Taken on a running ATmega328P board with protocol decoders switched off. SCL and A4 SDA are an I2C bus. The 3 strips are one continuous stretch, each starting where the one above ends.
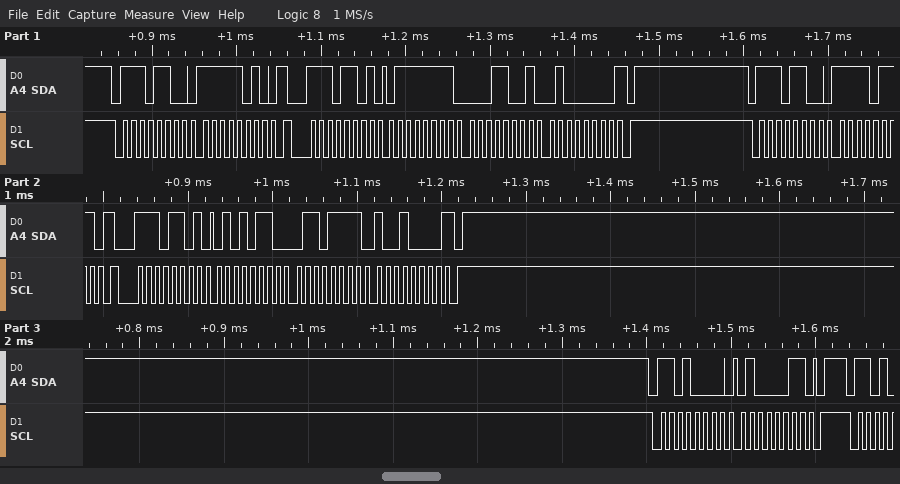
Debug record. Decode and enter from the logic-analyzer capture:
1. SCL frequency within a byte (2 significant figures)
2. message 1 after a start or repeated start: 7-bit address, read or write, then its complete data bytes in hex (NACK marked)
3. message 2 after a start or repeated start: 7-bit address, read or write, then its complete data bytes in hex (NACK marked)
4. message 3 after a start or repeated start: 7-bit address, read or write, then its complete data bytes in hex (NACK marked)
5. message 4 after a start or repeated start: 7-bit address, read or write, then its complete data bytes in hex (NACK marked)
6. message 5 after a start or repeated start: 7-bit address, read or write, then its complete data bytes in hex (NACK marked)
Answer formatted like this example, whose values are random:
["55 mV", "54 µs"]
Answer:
["100 kHz", "0x76 write: FA", "0x76 read: 7F 19 40 NACK", "0x76 write: F7", "0x76 read: 56 6F 90 NACK", "0x68 write: 43"]
